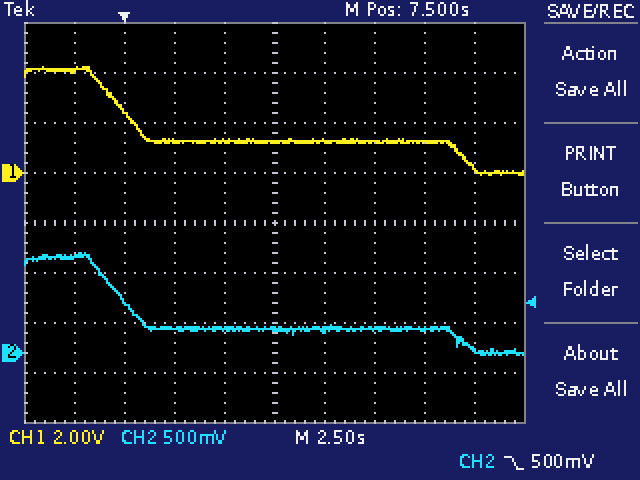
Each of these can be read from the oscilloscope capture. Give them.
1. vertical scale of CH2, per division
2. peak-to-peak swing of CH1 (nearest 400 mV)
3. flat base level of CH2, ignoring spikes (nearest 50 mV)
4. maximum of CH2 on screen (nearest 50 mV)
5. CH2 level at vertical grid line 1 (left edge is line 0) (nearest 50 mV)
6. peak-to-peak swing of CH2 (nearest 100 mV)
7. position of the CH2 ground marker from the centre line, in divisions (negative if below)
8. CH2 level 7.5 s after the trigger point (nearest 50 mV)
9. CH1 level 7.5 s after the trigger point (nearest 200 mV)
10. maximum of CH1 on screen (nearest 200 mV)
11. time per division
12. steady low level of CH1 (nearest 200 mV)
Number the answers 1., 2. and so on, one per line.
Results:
1. 500 mV
2. 4.4 V
3. 250 mV
4. 1.00 V
5. 950 mV
6. 1.00 V
7. -2.6 div
8. 250 mV
9. 1.2 V
10. 4.2 V
11. 2.5 s
12. 1.2 V
